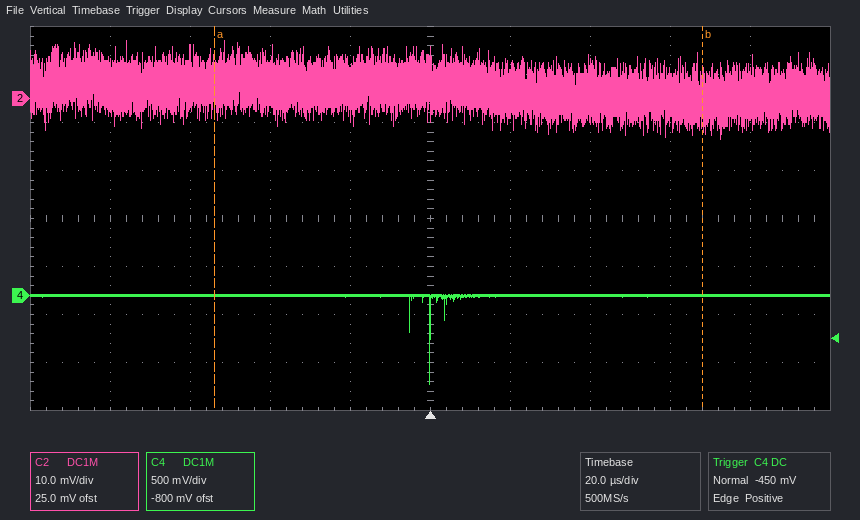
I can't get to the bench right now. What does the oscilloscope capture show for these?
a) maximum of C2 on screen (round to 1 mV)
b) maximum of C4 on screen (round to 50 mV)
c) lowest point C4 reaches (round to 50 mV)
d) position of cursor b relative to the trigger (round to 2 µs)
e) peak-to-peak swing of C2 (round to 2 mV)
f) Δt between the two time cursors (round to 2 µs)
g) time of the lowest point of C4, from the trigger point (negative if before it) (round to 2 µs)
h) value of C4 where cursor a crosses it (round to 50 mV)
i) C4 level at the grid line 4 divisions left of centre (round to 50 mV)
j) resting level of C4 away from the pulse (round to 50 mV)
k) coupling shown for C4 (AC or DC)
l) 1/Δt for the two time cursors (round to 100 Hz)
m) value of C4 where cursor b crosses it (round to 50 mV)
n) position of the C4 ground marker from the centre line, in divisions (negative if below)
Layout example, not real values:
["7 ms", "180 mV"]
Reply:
["12 mV", "0 mV", "-900 mV", "+68 µs", "20 mV", "122 µs", "0 µs", "0 mV", "0 mV", "0 mV", "DC", "8.2 kHz", "0 mV", "-1.6 div"]
